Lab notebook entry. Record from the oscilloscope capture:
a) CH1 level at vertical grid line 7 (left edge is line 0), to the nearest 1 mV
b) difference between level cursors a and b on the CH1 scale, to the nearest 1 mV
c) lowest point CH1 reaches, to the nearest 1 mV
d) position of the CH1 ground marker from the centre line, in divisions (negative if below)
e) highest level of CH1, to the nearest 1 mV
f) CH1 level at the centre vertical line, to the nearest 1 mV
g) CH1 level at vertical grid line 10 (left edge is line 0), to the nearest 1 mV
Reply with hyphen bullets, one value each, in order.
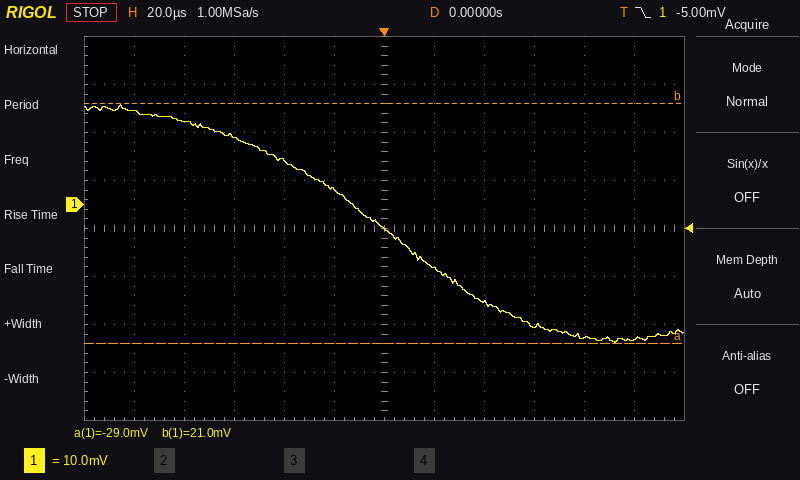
- -13 mV
- 50 mV
- -29 mV
- +0.5 div
- 21 mV
- -5 mV
- -28 mV
